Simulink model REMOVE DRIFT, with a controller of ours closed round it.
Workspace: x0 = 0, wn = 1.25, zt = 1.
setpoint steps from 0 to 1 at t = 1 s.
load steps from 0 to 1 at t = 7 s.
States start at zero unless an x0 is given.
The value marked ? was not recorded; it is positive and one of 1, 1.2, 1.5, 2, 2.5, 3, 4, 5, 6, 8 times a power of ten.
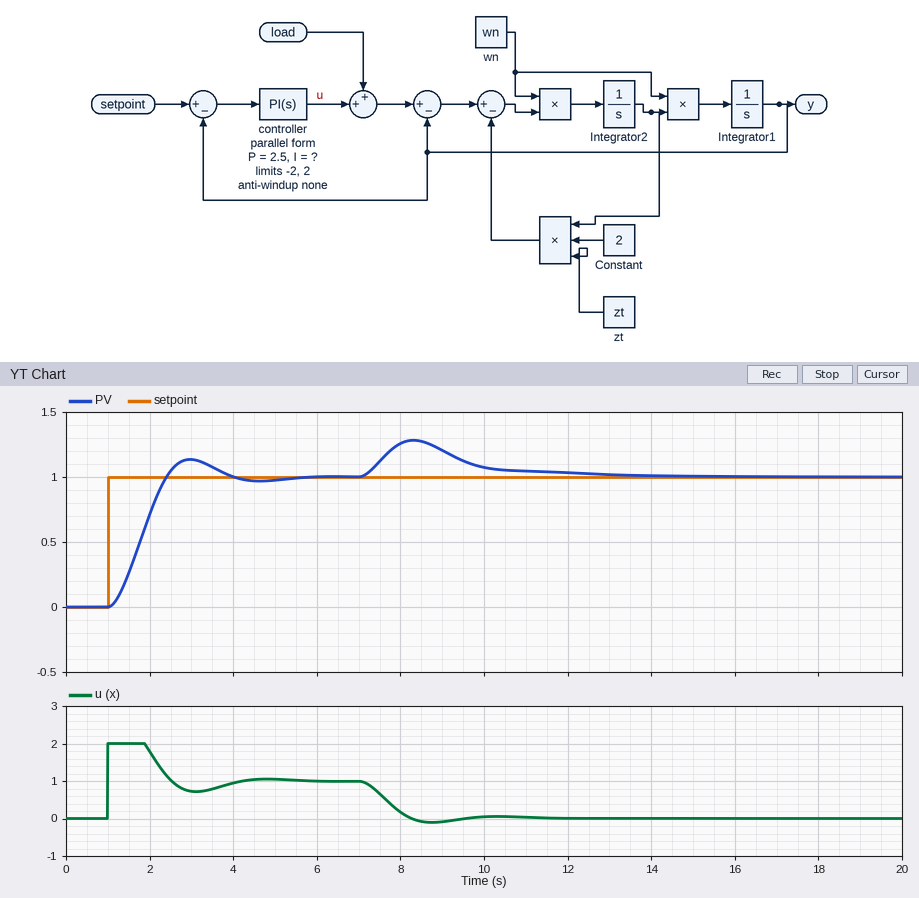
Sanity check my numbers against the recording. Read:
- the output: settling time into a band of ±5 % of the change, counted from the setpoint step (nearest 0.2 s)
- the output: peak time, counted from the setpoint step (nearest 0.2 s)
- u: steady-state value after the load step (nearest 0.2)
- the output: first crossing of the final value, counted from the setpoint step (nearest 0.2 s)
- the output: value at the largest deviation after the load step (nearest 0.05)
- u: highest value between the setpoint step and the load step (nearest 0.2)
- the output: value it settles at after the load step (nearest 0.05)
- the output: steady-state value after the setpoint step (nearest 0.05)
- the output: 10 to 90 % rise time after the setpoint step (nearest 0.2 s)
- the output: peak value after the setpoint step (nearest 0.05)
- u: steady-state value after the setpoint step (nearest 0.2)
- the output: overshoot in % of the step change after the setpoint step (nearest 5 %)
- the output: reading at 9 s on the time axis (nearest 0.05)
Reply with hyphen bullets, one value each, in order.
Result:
- 2.6 s
- 2.0 s
- 0.0
- 1.4 s
- 1.30
- 2.0
- 1.00
- 1.00
- 1.0 s
- 1.15
- 1.0
- 15 %
- 1.20
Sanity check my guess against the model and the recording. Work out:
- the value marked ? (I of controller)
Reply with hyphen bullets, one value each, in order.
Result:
- 1.5
